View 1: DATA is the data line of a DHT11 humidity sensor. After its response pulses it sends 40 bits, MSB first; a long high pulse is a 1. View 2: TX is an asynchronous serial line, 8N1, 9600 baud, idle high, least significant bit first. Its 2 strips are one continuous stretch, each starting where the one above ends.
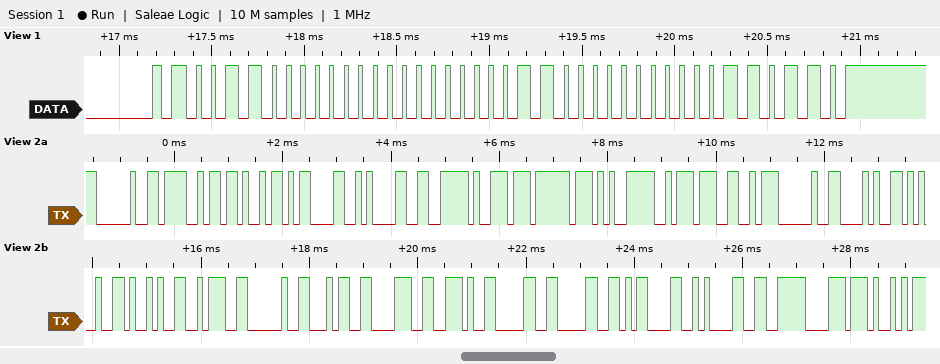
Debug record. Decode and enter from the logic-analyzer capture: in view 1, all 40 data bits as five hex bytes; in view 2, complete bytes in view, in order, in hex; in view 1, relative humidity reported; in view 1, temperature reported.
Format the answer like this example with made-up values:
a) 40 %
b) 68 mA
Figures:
a) 30 00 06 00 36
b) 0x20 0x4F 0x4B 0x0D 0x0A 0xE6 0xB9 0xBF 0xE5 0xBA 0xA6 0x20 0x28 0x25 0x29 0x3A 0x20 0x34 0x38 0x2E 0x30 0x30 0x0D 0x0A 0xE6 0xB8 0xA9
c) 48 %
d) 6.0 °C
